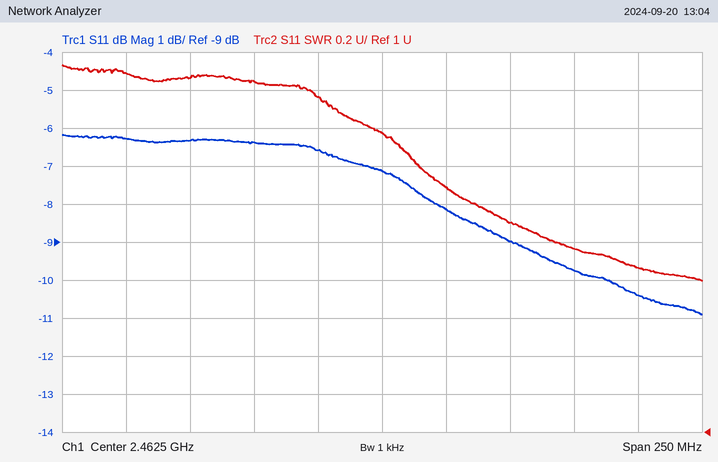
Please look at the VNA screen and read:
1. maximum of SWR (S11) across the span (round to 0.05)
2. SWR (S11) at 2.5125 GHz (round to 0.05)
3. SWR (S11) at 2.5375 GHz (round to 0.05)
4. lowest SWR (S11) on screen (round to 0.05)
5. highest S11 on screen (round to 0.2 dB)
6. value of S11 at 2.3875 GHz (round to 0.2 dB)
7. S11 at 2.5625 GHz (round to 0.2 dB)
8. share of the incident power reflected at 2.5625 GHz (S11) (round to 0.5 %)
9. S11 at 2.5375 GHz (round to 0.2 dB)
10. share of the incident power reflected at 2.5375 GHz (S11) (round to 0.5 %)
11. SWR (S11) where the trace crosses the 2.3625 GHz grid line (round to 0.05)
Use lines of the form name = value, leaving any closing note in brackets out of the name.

maximum of SWR (S11) across the span = 2.95
SWR (S11) at 2.5125 GHz = 2.10
SWR (S11) at 2.5375 GHz = 1.95
lowest SWR (S11) on screen = 1.80
highest S11 on screen = -6.2 dB
value of S11 at 2.3875 GHz = -6.4 dB
S11 at 2.5625 GHz = -10.4 dB
share of the incident power reflected at 2.5625 GHz (S11) = 9.0 %
S11 at 2.5375 GHz = -9.8 dB
share of the incident power reflected at 2.5375 GHz (S11) = 10.5 %
SWR (S11) where the trace crosses the 2.3625 GHz grid line = 2.90
